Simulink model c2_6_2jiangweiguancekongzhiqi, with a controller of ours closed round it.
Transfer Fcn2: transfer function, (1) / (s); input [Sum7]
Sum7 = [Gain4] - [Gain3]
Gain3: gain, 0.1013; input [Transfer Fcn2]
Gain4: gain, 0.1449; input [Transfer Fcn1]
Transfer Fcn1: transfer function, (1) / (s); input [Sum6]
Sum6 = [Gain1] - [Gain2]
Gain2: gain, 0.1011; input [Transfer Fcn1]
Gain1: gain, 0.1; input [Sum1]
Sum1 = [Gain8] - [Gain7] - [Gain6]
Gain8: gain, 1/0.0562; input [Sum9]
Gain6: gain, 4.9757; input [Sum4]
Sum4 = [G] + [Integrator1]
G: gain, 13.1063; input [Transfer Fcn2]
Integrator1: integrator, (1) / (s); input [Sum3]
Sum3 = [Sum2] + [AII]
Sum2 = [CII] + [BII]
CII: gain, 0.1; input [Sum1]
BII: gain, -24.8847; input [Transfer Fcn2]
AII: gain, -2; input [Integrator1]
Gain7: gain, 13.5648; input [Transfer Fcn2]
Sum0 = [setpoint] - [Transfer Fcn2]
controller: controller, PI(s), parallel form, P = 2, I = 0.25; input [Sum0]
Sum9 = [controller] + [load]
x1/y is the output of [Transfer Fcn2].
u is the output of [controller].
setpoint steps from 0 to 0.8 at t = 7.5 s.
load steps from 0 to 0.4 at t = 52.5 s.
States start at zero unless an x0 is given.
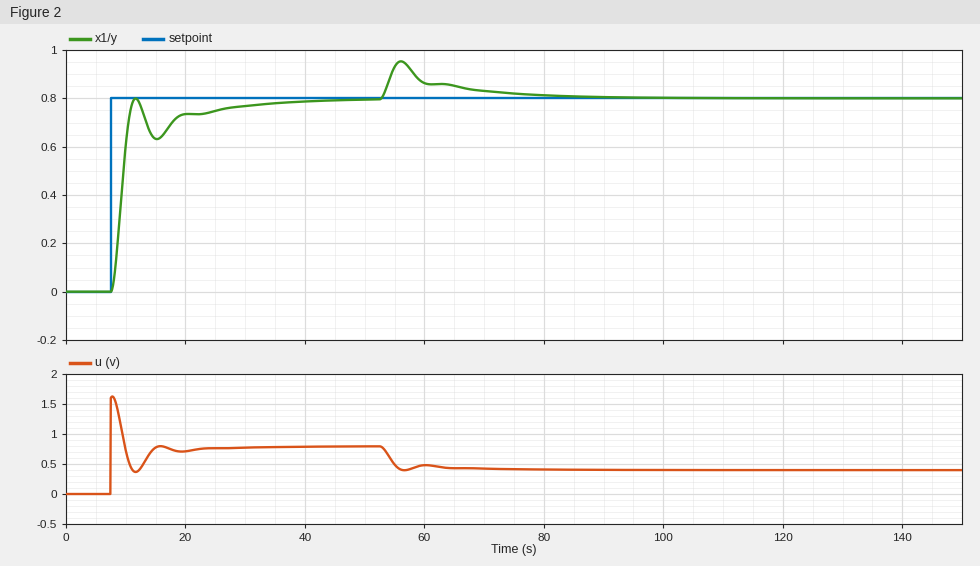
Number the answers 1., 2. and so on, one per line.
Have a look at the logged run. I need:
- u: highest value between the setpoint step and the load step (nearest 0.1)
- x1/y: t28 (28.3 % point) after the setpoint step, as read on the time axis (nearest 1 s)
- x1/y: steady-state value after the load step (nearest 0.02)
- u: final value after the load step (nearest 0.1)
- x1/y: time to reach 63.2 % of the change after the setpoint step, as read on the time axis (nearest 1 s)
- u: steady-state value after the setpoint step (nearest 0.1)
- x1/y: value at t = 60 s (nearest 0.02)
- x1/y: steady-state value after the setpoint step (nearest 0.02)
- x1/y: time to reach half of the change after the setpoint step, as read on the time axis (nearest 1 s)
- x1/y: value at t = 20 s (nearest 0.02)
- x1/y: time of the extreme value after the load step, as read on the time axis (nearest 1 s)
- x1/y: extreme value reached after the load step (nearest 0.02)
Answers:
1. 1.6
2. 9 s
3. 0.80
4. 0.4
5. 10 s
6. 0.8
7. 0.86
8. 0.80
9. 9 s
10. 0.74
11. 56 s
12. 0.96
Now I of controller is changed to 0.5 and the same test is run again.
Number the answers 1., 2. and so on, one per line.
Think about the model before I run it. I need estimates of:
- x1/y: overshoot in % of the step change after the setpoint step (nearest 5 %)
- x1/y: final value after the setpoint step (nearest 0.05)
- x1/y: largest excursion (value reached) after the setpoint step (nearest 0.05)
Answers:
1. 15 %
2. 0.80
3. 0.90
